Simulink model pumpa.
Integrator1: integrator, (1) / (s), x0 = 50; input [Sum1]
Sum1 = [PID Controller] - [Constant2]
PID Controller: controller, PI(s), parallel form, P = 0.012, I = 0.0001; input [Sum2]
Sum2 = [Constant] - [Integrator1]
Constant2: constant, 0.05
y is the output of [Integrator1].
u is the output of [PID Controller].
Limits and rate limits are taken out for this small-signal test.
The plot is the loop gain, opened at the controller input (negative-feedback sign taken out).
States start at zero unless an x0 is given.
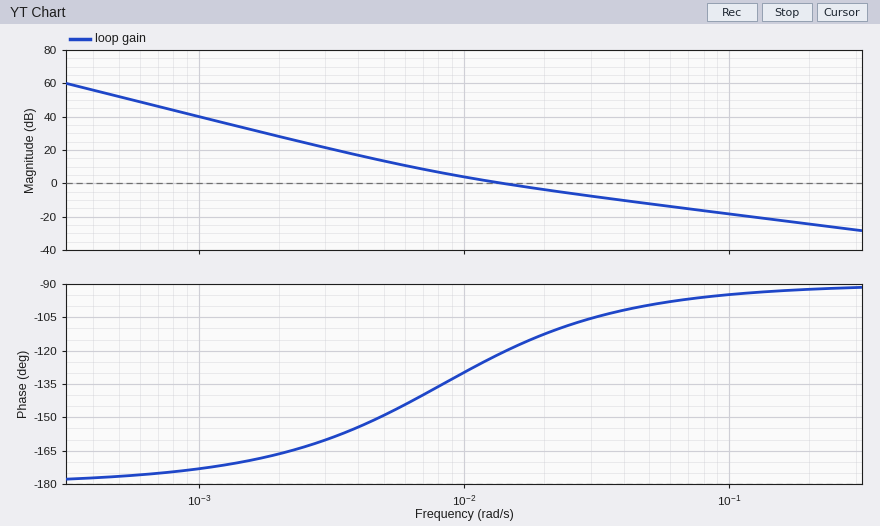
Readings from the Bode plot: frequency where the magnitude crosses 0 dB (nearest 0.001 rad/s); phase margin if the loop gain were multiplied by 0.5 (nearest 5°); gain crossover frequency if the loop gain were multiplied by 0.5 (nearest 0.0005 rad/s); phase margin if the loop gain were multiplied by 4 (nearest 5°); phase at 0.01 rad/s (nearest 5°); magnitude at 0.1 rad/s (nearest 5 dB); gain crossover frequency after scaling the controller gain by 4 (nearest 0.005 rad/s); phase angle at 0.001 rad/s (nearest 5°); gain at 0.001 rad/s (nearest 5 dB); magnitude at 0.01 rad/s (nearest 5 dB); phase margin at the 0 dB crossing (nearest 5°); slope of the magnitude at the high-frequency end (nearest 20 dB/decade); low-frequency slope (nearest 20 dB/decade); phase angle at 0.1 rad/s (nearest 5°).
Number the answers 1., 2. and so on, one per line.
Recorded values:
1. 0.014 rad/s
2. 45°
3. 0.0085 rad/s
4. 80°
5. -130°
6. -20 dB
7. 0.050 rad/s
8. -175°
9. 40 dB
10. 5 dB
11. 60°
12. -20 dB/decade
13. -40 dB/decade
14. -95°
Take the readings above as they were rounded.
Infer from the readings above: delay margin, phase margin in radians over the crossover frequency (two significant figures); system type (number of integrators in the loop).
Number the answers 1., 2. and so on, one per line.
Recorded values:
1. 75 s
2. 2
